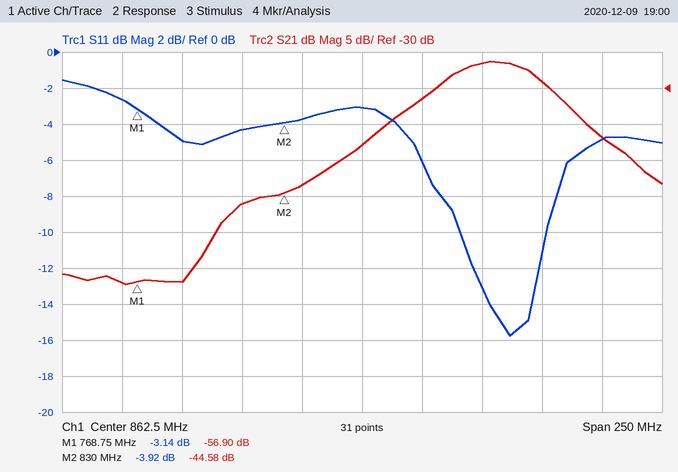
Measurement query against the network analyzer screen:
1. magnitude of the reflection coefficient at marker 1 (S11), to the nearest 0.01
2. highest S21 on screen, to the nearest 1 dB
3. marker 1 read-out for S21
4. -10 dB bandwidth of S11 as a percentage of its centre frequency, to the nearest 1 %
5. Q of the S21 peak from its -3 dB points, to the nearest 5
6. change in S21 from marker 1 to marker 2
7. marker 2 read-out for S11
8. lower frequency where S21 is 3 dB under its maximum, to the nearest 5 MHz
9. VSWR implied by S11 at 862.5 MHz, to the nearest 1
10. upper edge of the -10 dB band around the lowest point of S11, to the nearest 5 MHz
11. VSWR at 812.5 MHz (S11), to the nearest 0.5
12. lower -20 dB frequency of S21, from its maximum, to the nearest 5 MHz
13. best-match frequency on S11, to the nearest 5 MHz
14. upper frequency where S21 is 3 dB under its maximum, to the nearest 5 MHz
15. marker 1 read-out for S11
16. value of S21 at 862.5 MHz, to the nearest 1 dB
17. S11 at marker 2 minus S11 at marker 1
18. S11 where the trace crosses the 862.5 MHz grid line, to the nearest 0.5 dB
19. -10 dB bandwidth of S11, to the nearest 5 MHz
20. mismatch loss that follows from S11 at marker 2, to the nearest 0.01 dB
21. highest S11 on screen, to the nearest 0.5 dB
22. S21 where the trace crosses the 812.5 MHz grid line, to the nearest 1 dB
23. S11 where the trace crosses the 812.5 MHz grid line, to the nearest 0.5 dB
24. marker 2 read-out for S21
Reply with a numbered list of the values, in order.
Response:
1. 0.70
2. -26 dB
3. -56.90 dB
4. 4 %
5. 20
6. 12.32 dB
7. -3.92 dB
8. 895 MHz
9. 6
10. 940 MHz
11. 4.0
12. 810 MHz
13. 925 MHz
14. 940 MHz
15. -3.14 dB
16. -38 dB
17. -0.78 dB
18. -3.0 dB
19. 35 MHz
20. 2.26 dB
21. -1.5 dB
22. -46 dB
23. -4.5 dB
24. -44.58 dB
